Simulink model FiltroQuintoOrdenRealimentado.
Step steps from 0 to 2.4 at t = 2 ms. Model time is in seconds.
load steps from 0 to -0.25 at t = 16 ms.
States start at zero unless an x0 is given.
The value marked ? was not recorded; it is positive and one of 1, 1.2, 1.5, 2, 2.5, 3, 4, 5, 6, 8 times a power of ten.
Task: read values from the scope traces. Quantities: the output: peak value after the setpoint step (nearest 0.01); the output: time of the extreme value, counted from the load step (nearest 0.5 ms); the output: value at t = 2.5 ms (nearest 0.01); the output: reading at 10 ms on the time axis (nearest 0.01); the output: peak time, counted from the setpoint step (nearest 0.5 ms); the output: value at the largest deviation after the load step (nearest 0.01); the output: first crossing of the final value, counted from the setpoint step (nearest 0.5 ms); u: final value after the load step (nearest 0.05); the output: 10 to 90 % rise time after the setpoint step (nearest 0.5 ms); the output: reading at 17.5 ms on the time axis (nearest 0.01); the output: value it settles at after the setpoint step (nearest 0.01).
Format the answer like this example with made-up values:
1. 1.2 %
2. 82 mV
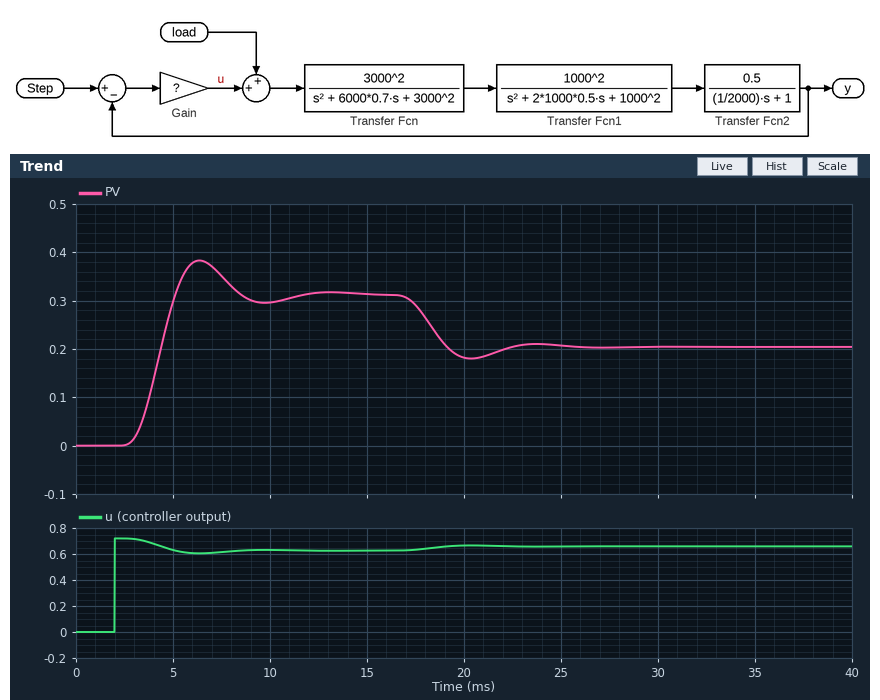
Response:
1. 0.38
2. 4.5 ms
3. 0.00
4. 0.30
5. 4.5 ms
6. 0.18
7. 3.0 ms
8. 0.65
9. 1.5 ms
10. 0.29
11. 0.31
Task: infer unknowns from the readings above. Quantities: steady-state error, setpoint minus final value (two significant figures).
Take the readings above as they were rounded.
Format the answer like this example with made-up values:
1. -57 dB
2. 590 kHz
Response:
1. 2.1
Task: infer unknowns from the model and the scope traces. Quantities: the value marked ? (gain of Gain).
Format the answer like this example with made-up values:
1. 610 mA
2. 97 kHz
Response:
1. 0.3
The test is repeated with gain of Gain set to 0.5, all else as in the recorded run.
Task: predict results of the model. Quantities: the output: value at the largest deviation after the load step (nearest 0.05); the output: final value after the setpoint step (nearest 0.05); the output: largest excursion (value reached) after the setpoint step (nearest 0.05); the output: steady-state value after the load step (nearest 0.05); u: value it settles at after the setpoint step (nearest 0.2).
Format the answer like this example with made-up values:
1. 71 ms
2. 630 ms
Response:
1. 0.35
2. 0.50
3. 0.60
4. 0.40
5. 1.0
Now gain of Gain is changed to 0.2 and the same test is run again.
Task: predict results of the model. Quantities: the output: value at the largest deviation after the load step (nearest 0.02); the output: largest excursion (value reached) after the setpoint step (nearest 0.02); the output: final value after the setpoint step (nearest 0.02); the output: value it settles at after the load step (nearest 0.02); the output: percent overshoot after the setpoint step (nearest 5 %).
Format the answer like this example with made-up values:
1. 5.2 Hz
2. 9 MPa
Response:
1. 0.08
2. 0.26
3. 0.22
4. 0.10
5. 20 %
